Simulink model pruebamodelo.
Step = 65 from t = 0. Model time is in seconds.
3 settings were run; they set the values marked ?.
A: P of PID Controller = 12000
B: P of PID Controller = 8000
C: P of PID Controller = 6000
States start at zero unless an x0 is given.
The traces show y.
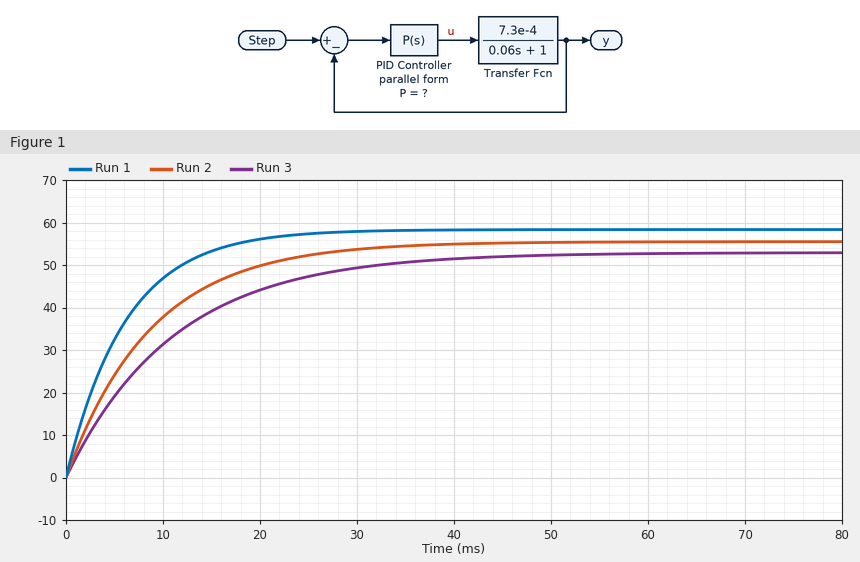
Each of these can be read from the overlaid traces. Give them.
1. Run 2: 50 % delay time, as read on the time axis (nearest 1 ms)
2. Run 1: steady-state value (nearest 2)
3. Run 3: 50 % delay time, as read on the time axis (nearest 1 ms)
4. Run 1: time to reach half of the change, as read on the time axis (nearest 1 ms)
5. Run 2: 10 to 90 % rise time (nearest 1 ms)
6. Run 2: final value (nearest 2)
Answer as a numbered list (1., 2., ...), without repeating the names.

1. 6 ms
2. 58
3. 8 ms
4. 4 ms
5. 19 ms
6. 56
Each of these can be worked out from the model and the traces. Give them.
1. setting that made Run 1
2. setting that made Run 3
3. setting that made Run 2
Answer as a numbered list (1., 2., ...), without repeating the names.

1. A
2. C
3. B
